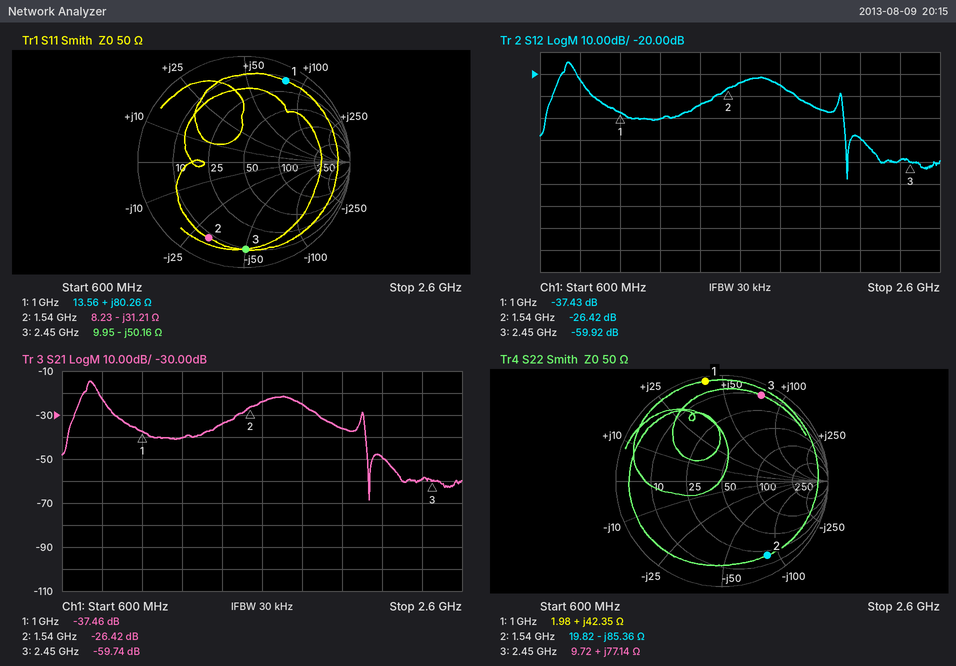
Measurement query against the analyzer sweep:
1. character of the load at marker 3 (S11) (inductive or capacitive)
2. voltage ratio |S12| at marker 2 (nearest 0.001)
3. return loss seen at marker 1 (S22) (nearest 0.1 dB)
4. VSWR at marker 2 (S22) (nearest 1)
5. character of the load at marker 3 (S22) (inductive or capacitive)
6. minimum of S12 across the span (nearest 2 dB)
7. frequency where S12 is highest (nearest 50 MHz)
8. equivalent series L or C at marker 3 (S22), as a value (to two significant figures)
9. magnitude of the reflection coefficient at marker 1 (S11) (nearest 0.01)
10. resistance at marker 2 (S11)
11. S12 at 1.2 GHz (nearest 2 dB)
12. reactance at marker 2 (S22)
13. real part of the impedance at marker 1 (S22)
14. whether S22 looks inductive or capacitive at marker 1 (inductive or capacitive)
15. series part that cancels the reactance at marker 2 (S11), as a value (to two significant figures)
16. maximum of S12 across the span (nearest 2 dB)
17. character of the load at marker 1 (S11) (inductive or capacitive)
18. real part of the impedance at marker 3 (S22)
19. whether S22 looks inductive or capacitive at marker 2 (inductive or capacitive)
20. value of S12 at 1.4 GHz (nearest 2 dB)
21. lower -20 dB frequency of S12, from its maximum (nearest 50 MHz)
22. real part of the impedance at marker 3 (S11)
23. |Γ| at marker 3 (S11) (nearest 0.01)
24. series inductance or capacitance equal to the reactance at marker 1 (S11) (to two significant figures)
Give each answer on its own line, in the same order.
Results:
capacitive
0.048
0.4 dB
10
inductive
-68 dB
750 MHz
5.0 nH
0.86
8.23 Ω
-40 dB
-85.36 Ω
1.98 Ω
inductive
3.2 nH
-14 dB
inductive
9.72 Ω
capacitive
-34 dB
650 MHz
9.95 Ω
0.82
13 nH
